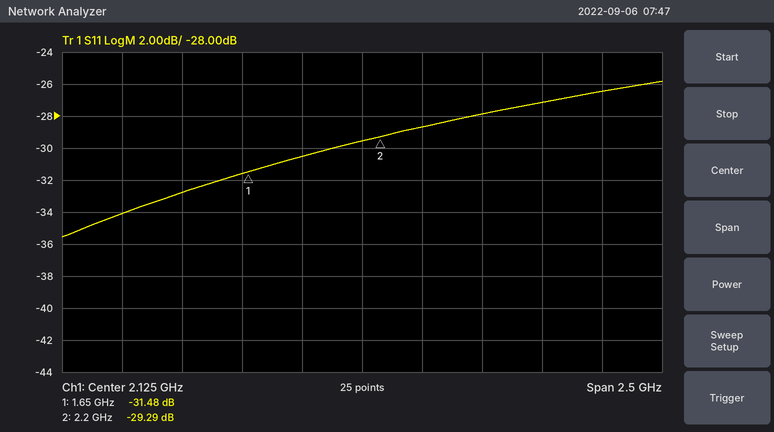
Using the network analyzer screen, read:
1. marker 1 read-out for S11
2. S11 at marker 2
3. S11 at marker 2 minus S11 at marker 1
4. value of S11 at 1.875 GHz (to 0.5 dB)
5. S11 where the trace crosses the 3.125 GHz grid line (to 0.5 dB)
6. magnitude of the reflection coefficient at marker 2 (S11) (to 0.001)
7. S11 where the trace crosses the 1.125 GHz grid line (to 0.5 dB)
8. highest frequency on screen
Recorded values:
-31.48 dB
-29.29 dB
2.19 dB
-30.5 dB
-26.5 dB
0.034
-34.0 dB
3.375 GHz
